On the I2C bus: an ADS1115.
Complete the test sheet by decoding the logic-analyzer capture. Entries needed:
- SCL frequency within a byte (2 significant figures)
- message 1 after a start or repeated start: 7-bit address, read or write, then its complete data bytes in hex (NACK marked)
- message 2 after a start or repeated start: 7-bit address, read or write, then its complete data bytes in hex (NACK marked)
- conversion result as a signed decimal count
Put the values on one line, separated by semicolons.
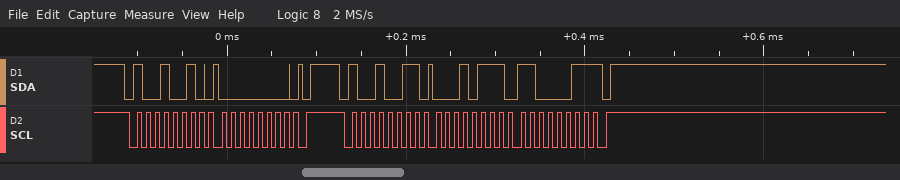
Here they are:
100 kHz; 0x49 write: 00; 0x49 read: 17 C3 NACK; 6083
